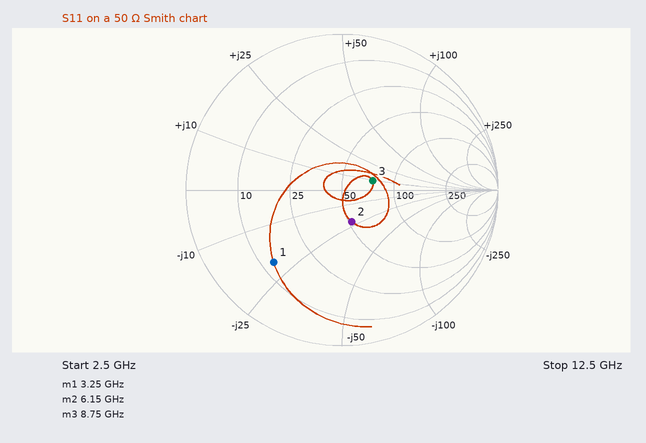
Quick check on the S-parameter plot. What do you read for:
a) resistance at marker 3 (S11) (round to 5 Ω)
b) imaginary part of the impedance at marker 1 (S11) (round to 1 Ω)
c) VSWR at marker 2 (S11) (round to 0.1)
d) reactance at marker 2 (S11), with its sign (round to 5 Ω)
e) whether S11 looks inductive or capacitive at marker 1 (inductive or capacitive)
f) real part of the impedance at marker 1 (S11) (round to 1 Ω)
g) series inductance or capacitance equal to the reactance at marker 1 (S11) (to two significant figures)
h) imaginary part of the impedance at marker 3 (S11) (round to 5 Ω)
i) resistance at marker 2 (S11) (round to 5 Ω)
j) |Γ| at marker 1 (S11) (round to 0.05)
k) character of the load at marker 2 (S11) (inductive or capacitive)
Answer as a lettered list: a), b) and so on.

a) 75 Ω
b) -20 Ω
c) 1.5
d) -20 Ω
e) capacitive
f) 13 Ω
g) 2.4 pF
h) +10 Ω
i) 50 Ω
j) 0.65
k) capacitive
